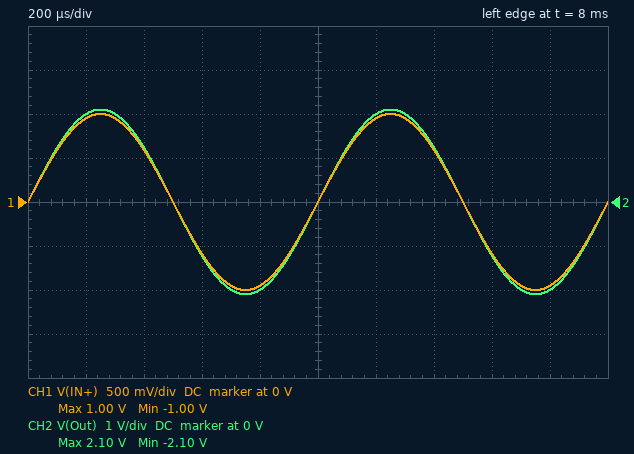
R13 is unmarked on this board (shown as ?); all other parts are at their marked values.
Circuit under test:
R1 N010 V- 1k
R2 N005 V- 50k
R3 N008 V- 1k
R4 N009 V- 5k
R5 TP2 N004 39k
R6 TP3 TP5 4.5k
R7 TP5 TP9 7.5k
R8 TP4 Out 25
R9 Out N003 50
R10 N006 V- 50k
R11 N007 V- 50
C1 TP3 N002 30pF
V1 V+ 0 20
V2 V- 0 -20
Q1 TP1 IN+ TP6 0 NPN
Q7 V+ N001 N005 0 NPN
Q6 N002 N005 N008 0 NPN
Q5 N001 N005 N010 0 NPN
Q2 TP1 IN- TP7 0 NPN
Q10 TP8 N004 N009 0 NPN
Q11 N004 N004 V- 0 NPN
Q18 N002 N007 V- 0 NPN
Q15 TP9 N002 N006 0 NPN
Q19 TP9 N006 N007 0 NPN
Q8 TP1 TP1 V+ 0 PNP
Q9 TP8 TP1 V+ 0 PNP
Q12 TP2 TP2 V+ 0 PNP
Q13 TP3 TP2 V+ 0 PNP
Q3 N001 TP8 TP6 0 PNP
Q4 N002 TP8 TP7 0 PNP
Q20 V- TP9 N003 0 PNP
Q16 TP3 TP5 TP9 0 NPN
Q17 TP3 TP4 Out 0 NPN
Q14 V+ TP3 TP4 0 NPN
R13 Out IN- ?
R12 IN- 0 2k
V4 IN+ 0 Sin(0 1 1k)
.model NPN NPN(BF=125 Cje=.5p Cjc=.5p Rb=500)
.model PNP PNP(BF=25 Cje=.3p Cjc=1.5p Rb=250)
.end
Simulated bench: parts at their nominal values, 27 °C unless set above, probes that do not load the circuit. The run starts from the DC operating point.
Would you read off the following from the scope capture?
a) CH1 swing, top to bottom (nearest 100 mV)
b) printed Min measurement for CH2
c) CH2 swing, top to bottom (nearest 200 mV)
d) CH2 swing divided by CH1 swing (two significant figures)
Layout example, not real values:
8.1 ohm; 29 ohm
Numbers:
2.0 V; -2.10 V; 4.2 V; 2.1
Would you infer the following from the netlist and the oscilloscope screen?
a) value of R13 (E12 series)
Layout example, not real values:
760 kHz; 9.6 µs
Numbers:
2.2 kΩ
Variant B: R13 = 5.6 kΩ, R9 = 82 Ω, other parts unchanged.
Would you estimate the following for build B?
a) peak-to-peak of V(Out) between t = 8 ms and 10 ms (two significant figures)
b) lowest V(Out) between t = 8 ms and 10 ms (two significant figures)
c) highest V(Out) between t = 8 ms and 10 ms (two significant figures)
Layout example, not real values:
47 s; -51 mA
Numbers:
7.6 V; -3.8 V; 3.8 V
